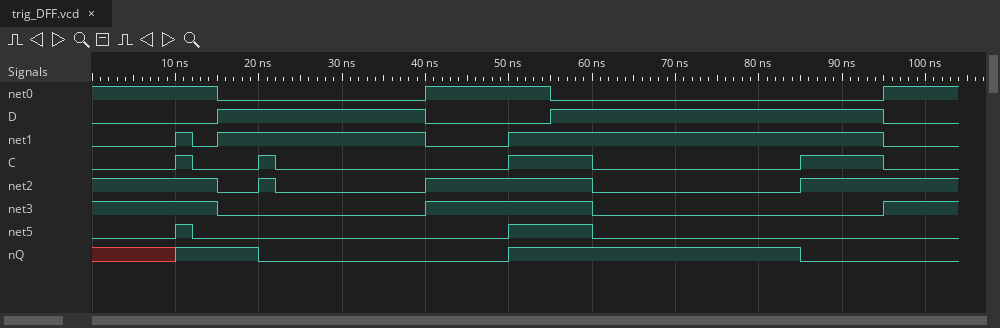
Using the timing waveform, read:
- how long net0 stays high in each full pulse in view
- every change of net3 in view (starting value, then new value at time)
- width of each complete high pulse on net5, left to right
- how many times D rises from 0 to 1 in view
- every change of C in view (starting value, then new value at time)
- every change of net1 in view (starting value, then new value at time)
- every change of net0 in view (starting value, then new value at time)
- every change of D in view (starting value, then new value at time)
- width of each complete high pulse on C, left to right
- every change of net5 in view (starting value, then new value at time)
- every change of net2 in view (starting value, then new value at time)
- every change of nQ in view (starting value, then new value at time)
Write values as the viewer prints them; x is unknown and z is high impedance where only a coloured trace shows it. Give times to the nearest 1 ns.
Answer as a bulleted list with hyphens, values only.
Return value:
- 15 ns
- 1, 0 at 15 ns, 1 at 40 ns, 0 at 60 ns, 1 at 95 ns
- 2 ns, 10 ns
- 2
- 0, 1 at 10 ns, 0 at 12 ns, 1 at 20 ns, 0 at 22 ns, 1 at 50 ns, 0 at 60 ns, 1 at 85 ns, 0 at 95 ns
- 0, 1 at 10 ns, 0 at 12 ns, 1 at 15 ns, 0 at 40 ns, 1 at 50 ns, 0 at 95 ns
- 1, 0 at 15 ns, 1 at 40 ns, 0 at 55 ns, 1 at 95 ns
- 0, 1 at 15 ns, 0 at 40 ns, 1 at 55 ns, 0 at 95 ns
- 2 ns, 2 ns, 10 ns, 10 ns
- 0, 1 at 10 ns, 0 at 12 ns, 1 at 50 ns, 0 at 60 ns
- 1, 0 at 15 ns, 1 at 20 ns, 0 at 22 ns, 1 at 40 ns, 0 at 60 ns, 1 at 85 ns
- x, 1 at 10 ns, 0 at 20 ns, 1 at 50 ns, 0 at 85 ns
